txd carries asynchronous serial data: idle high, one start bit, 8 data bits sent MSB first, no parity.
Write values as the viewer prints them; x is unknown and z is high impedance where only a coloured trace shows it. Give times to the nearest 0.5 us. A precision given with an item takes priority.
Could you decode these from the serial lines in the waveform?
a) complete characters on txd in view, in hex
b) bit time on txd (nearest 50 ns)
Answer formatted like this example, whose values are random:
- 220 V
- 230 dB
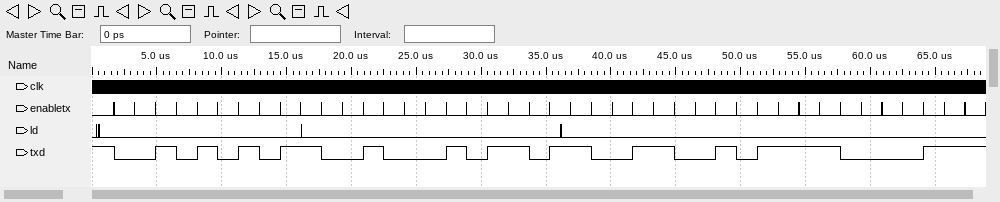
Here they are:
- 55, 45, CC, F0
- 1600 ns
